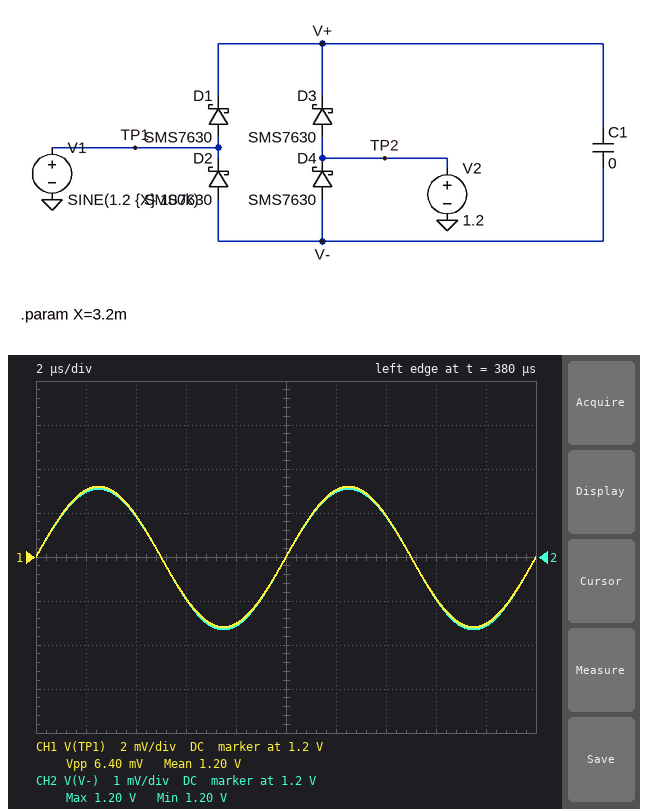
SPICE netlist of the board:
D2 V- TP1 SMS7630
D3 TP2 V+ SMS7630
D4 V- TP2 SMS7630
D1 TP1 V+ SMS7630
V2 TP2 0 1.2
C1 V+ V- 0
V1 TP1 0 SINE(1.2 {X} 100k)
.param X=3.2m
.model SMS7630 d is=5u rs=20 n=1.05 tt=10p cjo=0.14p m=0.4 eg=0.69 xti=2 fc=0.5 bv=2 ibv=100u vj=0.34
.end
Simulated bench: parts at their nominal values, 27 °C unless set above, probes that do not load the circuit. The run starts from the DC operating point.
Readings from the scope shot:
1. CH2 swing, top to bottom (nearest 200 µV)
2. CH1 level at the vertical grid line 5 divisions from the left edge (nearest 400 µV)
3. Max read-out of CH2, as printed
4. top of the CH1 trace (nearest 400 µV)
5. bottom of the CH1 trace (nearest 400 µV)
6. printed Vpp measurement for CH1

3.2 mV
1.2000 V
1.20 V
1.2032 V
1.1968 V
6.40 mV
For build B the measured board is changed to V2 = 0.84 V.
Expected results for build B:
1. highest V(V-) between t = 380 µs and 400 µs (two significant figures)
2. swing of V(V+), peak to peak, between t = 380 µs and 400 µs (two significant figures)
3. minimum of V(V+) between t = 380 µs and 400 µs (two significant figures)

860 mV
6.4 mV
1.2 V
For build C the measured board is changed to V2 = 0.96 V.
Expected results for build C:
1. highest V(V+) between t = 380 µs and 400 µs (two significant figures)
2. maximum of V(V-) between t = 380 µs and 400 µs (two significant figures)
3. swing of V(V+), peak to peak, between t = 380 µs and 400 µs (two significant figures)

1.2 V
980 mV
6.4 mV
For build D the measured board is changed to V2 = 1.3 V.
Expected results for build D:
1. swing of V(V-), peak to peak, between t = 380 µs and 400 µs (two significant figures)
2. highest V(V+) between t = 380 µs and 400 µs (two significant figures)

6.2 mV
1.3 V
